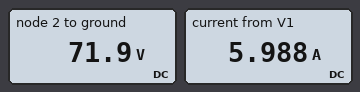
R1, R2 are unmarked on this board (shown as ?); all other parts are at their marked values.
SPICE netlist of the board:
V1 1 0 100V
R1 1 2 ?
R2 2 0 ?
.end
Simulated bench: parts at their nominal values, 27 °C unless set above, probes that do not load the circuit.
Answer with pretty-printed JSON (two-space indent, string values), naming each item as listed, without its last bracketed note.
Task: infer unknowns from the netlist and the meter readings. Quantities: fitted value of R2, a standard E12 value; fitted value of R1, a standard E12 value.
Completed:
{
  "fitted value of R2, a standard E12 value": "12 Ω",
  "fitted value of R1, a standard E12 value": "4.7 Ω"
}
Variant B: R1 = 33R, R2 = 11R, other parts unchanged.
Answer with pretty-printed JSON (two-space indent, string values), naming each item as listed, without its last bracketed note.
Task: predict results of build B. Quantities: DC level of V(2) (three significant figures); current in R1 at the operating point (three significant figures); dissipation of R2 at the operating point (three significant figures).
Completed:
{
  "DC level of V(2)": "25.0 V",
  "current in R1 at the operating point": "2.27 A",
  "dissipation of R2 at the operating point": "56.8 W"
}
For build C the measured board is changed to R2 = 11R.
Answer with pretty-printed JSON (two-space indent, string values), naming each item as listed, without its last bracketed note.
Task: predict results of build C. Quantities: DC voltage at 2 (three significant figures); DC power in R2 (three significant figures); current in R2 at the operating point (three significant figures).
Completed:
{
  "DC voltage at 2": "70.1 V",
  "DC power in R2": "446 W",
  "current in R2 at the operating point": "6.37 A"
}
